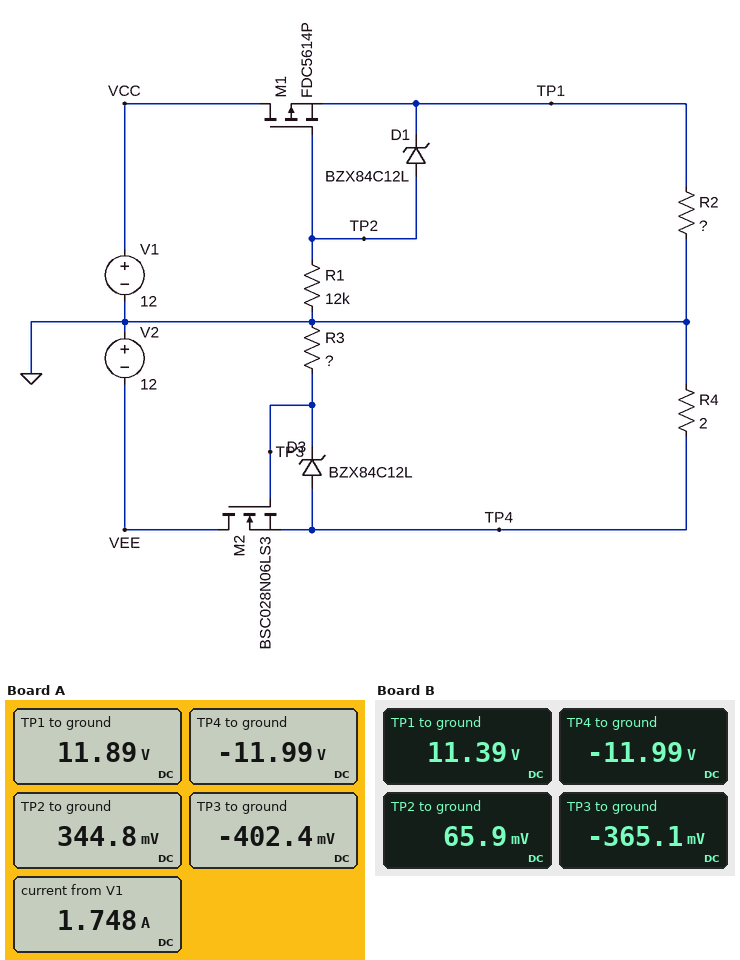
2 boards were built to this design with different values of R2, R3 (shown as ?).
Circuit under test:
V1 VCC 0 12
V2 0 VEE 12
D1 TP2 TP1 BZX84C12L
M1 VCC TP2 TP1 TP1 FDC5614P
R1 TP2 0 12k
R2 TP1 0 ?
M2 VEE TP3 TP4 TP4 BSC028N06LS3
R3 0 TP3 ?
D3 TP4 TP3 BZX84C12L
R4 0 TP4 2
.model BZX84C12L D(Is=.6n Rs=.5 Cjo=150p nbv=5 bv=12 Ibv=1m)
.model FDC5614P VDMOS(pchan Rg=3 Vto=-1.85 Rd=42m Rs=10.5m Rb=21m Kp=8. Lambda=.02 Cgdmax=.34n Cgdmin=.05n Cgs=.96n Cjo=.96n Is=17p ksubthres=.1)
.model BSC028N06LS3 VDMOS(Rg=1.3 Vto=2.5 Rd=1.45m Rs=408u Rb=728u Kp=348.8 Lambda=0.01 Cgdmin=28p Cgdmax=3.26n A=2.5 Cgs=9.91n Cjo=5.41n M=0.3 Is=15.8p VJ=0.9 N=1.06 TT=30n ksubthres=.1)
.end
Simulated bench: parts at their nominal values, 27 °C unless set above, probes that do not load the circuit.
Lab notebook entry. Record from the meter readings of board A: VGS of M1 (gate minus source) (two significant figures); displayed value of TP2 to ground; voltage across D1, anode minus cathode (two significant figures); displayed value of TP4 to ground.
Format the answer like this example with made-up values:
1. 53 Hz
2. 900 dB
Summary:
1. -12 V
2. 344.8 mV
3. -12 V
4. -11.99 V
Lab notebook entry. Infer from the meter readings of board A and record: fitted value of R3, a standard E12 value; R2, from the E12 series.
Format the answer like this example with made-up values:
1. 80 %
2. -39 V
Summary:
1. 10 kΩ
2. 6.8 Ω
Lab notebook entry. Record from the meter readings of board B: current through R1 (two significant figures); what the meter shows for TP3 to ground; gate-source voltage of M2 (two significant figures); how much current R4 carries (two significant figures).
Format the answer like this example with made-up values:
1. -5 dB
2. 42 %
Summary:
1. 5.5 µA
2. -365.1 mV
3. 12 V
4. 6.0 A
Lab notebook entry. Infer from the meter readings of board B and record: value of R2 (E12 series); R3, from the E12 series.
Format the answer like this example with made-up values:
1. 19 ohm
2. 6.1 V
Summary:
1. 1.2 Ω
2. 6.8 kΩ
